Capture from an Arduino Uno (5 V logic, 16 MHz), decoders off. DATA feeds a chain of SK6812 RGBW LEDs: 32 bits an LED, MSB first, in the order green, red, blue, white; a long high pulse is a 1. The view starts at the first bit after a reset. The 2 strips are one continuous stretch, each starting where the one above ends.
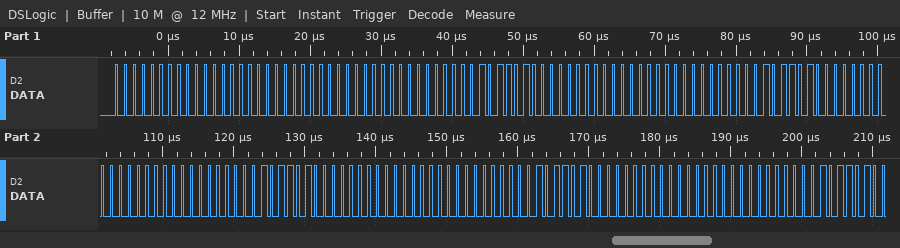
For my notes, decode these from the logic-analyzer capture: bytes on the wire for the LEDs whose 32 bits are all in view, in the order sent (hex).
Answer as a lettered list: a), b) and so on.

a) 00 00 00 00 00 5A 00 00 00 5A 00 00 00 5A 00 00 00 B4 00 00
